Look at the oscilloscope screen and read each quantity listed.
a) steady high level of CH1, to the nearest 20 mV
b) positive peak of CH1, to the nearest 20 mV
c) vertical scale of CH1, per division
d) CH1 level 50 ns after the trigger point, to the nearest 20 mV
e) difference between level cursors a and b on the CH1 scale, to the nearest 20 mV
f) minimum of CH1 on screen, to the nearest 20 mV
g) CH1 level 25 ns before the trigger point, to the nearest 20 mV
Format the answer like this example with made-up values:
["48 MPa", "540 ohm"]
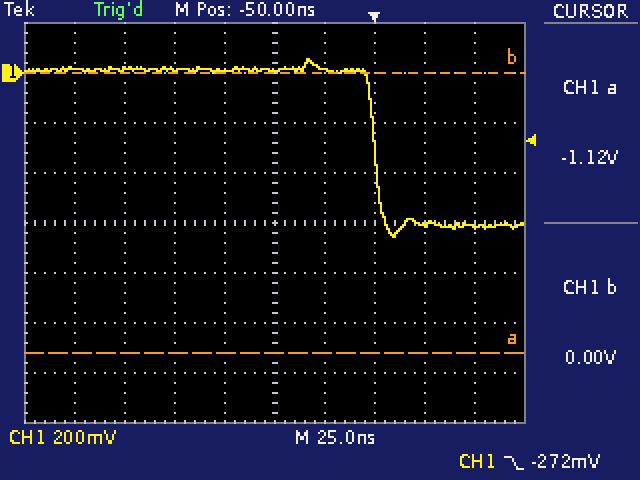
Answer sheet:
["20 mV", "60 mV", "200 mV", "-620 mV", "1.12 V", "-660 mV", "20 mV"]
